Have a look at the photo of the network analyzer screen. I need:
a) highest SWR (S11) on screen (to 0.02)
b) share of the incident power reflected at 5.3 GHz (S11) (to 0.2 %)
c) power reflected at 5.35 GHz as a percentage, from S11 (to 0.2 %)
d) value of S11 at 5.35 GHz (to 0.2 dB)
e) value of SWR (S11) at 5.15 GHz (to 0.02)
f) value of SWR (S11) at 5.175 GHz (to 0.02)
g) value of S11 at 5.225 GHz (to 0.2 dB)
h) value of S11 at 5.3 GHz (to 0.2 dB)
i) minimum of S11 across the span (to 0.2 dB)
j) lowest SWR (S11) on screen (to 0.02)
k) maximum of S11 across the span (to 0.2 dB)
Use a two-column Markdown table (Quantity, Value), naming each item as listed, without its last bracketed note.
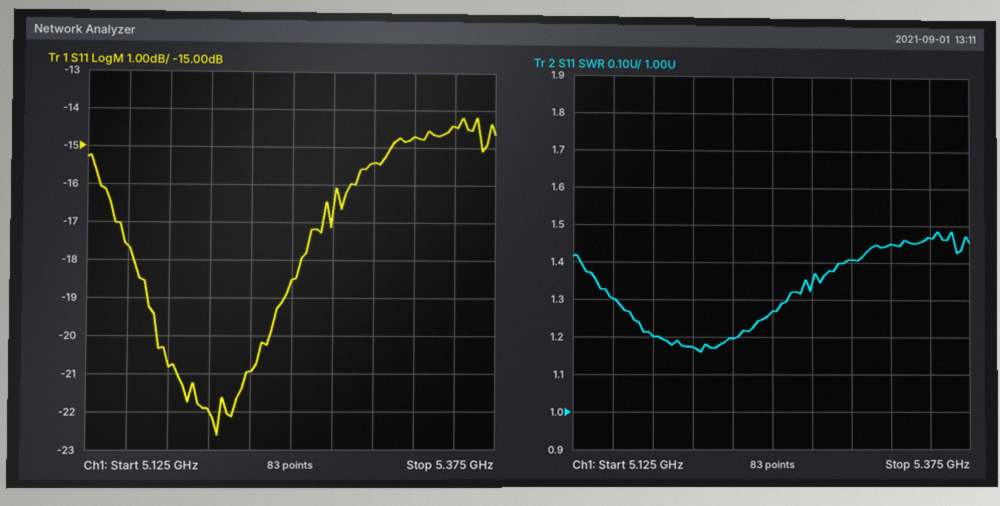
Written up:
| Quantity | Value |
|---|---|
| highest SWR (S11) on screen | 1.48 |
| share of the incident power reflected at 5.3 GHz (S11) | 2.8 % |
| power reflected at 5.35 GHz as a percentage, from S11 | 3.6 % |
| value of S11 at 5.35 GHz | -14.4 dB |
| value of SWR (S11) at 5.15 GHz | 1.30 |
| value of SWR (S11) at 5.175 GHz | 1.20 |
| value of S11 at 5.225 GHz | -21.0 dB |
| value of S11 at 5.3 GHz | -15.4 dB |
| minimum of S11 across the span | -22.6 dB |
| lowest SWR (S11) on screen | 1.16 |
| maximum of S11 across the span | -14.2 dB |
